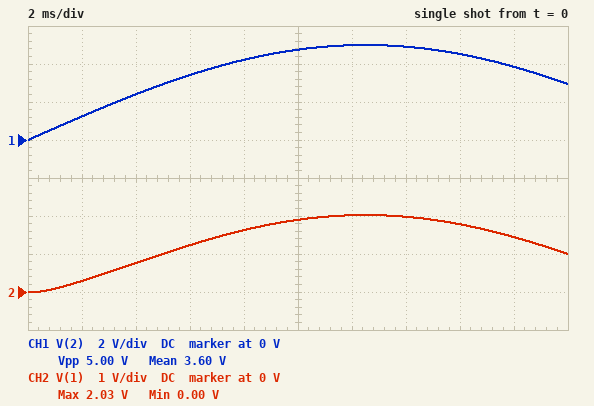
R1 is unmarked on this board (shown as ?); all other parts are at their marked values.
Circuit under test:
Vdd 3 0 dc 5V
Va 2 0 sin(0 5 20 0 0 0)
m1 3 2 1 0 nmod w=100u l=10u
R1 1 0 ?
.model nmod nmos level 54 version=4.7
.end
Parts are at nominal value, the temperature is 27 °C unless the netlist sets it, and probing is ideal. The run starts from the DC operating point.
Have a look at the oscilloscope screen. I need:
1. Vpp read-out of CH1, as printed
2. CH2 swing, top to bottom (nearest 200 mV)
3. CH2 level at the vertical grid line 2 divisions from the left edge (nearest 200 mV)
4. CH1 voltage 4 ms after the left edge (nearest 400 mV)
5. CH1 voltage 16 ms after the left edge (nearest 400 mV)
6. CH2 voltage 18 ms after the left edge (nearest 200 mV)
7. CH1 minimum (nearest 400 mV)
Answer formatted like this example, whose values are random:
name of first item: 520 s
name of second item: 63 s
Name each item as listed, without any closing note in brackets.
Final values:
Vpp read-out of CH1, as printed: 5.00 V
CH2 swing, top to bottom: 2.0 V
CH2 level at the vertical grid line 2 divisions from the left edge: 800 mV
CH1 voltage 4 ms after the left edge: 2.4 V
CH1 voltage 16 ms after the left edge: 4.4 V
CH2 voltage 18 ms after the left edge: 1.4 V
CH1 minimum: 0 V
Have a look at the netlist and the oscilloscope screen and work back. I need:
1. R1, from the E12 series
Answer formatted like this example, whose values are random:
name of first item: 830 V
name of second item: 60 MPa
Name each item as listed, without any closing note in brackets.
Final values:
R1, from the E12 series: 180 Ω
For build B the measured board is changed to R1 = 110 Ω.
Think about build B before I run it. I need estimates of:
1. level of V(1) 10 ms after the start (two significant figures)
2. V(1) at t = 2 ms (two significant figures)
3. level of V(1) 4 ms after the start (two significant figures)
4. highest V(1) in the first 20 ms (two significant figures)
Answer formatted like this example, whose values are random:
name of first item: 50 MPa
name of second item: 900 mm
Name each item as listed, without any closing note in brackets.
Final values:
level of V(1) 10 ms after the start: 1.5 V
V(1) at t = 2 ms: 210 mV
level of V(1) 4 ms after the start: 580 mV
highest V(1) in the first 20 ms: 1.6 V
